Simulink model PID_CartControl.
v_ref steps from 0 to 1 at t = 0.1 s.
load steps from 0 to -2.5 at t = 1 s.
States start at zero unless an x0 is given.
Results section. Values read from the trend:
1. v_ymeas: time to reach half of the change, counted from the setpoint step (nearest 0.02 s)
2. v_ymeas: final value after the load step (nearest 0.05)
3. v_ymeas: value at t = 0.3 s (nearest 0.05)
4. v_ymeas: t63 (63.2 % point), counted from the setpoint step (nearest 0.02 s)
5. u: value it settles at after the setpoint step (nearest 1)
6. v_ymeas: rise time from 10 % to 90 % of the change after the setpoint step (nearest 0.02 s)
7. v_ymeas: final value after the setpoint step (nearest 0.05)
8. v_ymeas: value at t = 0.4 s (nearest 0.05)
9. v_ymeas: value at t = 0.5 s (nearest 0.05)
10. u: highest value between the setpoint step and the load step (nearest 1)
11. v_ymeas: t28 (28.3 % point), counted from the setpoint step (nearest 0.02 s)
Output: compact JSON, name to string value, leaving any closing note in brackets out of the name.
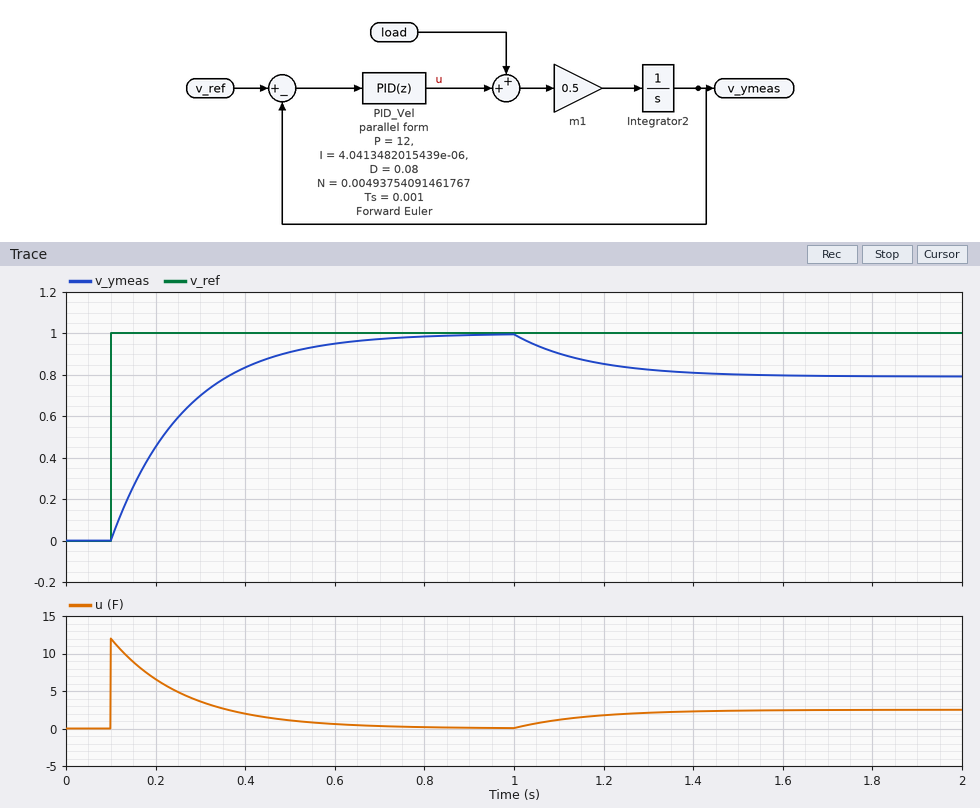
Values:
{"v_ymeas: time to reach half of the change, counted from the setpoint step": "0.12 s", "v_ymeas: final value after the load step": "0.80", "v_ymeas: value at t = 0.3 s": "0.70", "v_ymeas: t63 (63.2 % point), counted from the setpoint step": "0.16 s", "u: value it settles at after the setpoint step": "0", "v_ymeas: rise time from 10 % to 90 % of the change after the setpoint step": "0.36 s", "v_ymeas: final value after the setpoint step": "1.00", "v_ymeas: value at t = 0.4 s": "0.85", "v_ymeas: value at t = 0.5 s": "0.90", "u: highest value between the setpoint step and the load step": "12", "v_ymeas: t28 (28.3 % point), counted from the setpoint step": "0.06 s"}
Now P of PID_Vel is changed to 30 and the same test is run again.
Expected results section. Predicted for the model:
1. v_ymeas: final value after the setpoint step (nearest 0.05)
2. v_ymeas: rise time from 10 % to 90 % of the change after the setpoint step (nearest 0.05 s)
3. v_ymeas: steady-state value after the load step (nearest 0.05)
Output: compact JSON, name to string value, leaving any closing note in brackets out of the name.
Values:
{"v_ymeas: final value after the setpoint step": "1.00", "v_ymeas: rise time from 10 % to 90 % of the change after the setpoint step": "0.15 s", "v_ymeas: steady-state value after the load step": "0.90"}
